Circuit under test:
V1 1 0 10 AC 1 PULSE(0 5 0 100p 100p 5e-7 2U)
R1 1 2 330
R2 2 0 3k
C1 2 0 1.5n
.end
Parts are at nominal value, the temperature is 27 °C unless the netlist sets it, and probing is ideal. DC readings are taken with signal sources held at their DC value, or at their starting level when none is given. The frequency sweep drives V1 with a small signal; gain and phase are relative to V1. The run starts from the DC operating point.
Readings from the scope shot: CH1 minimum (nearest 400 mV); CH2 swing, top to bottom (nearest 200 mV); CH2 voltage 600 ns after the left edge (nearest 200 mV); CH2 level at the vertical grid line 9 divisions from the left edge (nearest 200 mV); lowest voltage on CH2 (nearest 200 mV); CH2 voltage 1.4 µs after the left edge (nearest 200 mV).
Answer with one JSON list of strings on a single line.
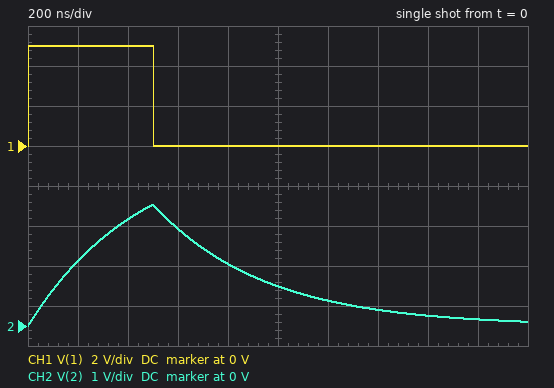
["0 V", "3.0 V", "2.4 V", "200 mV", "0 V", "400 mV"]
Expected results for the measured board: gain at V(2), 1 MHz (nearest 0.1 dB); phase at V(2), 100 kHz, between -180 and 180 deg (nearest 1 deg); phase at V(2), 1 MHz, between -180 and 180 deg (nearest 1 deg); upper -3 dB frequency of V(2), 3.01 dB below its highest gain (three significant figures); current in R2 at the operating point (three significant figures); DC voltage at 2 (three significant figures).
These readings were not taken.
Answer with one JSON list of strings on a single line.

["-10.4 dB", "-16 deg", "-70 deg", "357 kHz", "3.00 mA", "9.01 V"]
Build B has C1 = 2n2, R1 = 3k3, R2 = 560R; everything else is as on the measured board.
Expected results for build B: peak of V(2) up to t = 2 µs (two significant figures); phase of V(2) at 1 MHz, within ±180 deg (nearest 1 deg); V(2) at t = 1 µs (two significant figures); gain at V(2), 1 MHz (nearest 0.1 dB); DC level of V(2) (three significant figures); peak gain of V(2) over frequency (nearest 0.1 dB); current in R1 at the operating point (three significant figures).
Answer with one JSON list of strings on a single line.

["270 mV", "-81 deg", "170 mV", "-33.3 dB", "1.45 V", "-16.8 dB", "2.59 mA"]
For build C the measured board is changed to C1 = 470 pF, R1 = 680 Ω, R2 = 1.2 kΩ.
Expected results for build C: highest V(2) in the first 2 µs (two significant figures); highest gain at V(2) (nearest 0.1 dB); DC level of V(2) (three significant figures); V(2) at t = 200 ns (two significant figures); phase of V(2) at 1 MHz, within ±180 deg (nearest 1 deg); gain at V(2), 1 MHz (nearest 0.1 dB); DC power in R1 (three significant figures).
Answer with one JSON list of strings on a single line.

["2.9 V", "-3.9 dB", "6.38 V", "2.0 V", "-52 deg", "-8.1 dB", "19.2 mW"]
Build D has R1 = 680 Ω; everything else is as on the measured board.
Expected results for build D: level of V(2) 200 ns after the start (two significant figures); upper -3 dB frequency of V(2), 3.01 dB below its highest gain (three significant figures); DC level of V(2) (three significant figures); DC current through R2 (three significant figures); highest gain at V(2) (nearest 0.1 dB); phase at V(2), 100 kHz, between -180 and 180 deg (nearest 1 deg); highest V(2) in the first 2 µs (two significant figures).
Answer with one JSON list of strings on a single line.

["870 mV", "191 kHz", "8.15 V", "2.72 mA", "-1.8 dB", "-28 deg", "1.8 V"]
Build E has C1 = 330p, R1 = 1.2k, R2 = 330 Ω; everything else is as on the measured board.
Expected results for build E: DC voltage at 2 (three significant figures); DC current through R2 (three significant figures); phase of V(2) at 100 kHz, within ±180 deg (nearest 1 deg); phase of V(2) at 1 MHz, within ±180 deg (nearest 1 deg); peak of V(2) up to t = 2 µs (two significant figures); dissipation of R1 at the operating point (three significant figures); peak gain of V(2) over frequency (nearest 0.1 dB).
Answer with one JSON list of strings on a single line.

["2.16 V", "6.54 mA", "-3 deg", "-28 deg", "1.1 V", "51.3 mW", "-13.3 dB"]
